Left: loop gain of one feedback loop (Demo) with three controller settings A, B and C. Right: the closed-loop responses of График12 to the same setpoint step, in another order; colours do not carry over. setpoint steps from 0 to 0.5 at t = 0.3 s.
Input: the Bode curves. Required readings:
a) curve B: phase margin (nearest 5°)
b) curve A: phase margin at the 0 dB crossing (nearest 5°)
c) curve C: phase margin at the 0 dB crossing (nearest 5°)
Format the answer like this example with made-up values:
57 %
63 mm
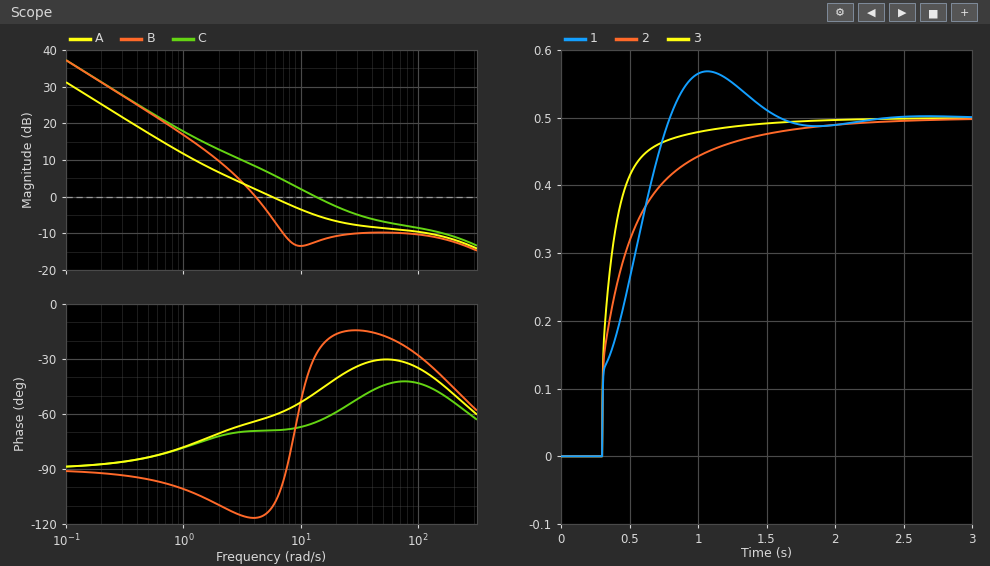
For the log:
65°
120°
115°
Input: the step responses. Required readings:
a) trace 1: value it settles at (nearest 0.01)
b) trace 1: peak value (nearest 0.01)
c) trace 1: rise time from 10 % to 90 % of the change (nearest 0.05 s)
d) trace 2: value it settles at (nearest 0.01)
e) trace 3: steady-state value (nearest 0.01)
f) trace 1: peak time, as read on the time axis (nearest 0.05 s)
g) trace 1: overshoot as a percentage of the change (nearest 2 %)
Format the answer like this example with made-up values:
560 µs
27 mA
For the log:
0.50
0.57
0.40 s
0.50
0.50
1.05 s
14 %
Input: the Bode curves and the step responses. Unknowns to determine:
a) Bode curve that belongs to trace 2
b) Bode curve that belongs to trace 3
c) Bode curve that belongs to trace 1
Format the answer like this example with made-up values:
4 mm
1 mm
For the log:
A
C
B
